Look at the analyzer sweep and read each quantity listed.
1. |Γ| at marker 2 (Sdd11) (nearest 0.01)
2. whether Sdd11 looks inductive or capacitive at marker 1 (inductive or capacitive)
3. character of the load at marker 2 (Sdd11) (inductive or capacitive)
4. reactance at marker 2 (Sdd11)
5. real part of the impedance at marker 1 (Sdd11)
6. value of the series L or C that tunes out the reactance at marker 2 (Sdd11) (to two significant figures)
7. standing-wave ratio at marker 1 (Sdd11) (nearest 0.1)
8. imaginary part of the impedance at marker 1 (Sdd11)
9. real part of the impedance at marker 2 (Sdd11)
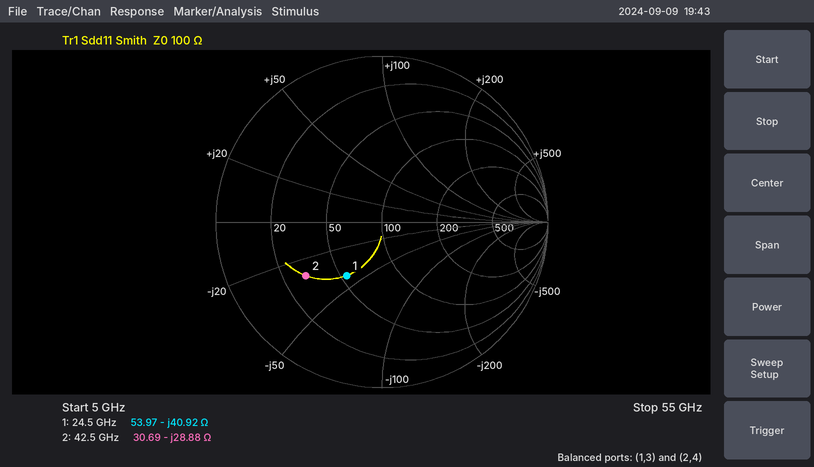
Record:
0.56
capacitive
capacitive
-28.88 Ω
53.97 Ω
110 pH
2.3
-40.92 Ω
30.69 Ω
